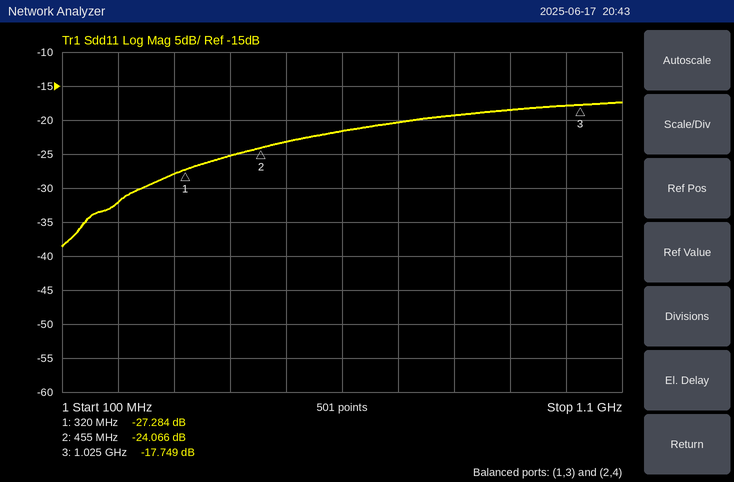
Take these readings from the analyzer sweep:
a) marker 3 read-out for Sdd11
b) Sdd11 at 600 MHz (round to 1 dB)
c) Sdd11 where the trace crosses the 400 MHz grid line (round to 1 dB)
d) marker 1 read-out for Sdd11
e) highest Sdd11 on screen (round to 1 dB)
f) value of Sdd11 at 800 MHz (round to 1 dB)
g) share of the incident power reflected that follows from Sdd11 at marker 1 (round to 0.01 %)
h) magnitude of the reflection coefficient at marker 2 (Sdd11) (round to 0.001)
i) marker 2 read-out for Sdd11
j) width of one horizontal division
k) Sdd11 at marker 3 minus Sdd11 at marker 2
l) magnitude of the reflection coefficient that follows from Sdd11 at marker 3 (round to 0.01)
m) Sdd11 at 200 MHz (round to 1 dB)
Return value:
-17.749 dB
-22 dB
-25 dB
-27.284 dB
-17 dB
-19 dB
0.19 %
0.063
-24.066 dB
100 MHz
6.317 dB
0.13
-32 dB
